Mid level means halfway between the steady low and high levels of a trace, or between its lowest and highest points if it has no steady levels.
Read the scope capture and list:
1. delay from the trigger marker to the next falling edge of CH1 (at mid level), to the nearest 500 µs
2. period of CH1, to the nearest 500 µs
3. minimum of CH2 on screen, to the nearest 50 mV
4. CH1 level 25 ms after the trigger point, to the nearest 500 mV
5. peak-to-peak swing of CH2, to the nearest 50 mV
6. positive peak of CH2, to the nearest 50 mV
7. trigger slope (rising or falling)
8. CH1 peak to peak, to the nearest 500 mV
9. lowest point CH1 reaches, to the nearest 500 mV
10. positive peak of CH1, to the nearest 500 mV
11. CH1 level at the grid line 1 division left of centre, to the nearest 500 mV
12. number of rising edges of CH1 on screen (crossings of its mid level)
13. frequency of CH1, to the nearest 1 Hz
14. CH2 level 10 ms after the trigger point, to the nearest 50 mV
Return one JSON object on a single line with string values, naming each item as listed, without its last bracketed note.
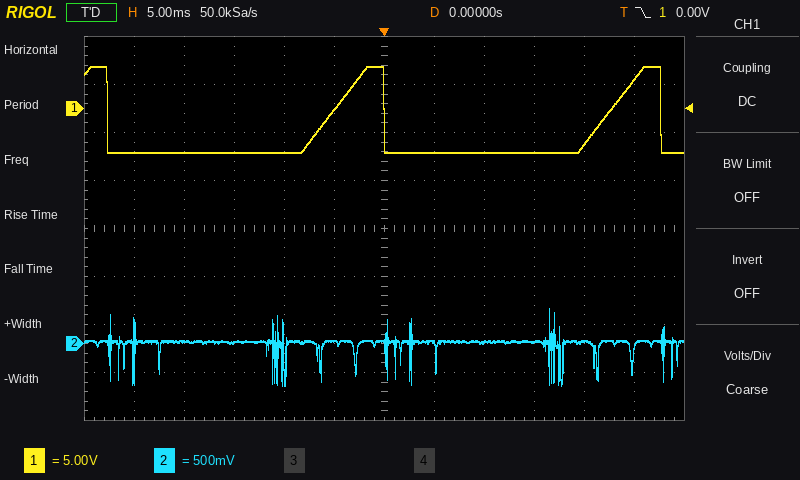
{"delay from the trigger marker to the next falling edge of CH1 (at mid level), to the nearest 500 µs": "27.5 ms", "period of CH1, to the nearest 500 µs": "27.5 ms", "minimum of CH2 on screen, to the nearest 50 mV": "-450 mV", "CH1 level 25 ms after the trigger point, to the nearest 500 mV": "3.0 V", "peak-to-peak swing of CH2, to the nearest 50 mV": "800 mV", "positive peak of CH2, to the nearest 50 mV": "350 mV", "trigger slope": "falling", "CH1 peak to peak, to the nearest 500 mV": "9.0 V", "lowest point CH1 reaches, to the nearest 500 mV": "-4.5 V", "positive peak of CH1, to the nearest 500 mV": "4.5 V", "CH1 level at the grid line 1 division left of centre, to the nearest 500 mV": "0.0 V", "number of rising edges of CH1 on screen": "2", "frequency of CH1, to the nearest 1 Hz": "36 Hz", "CH2 level 10 ms after the trigger point, to the nearest 50 mV": "0 mV"}
